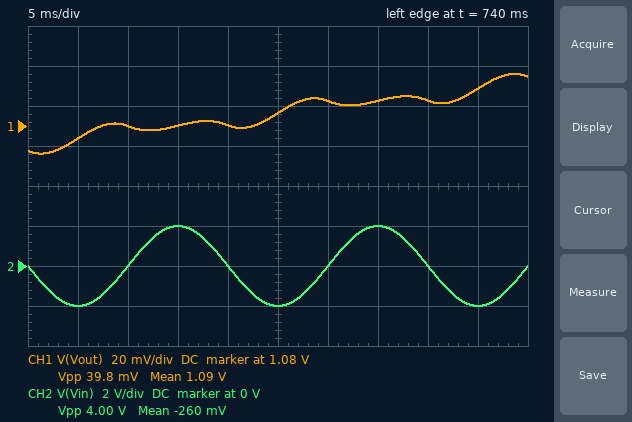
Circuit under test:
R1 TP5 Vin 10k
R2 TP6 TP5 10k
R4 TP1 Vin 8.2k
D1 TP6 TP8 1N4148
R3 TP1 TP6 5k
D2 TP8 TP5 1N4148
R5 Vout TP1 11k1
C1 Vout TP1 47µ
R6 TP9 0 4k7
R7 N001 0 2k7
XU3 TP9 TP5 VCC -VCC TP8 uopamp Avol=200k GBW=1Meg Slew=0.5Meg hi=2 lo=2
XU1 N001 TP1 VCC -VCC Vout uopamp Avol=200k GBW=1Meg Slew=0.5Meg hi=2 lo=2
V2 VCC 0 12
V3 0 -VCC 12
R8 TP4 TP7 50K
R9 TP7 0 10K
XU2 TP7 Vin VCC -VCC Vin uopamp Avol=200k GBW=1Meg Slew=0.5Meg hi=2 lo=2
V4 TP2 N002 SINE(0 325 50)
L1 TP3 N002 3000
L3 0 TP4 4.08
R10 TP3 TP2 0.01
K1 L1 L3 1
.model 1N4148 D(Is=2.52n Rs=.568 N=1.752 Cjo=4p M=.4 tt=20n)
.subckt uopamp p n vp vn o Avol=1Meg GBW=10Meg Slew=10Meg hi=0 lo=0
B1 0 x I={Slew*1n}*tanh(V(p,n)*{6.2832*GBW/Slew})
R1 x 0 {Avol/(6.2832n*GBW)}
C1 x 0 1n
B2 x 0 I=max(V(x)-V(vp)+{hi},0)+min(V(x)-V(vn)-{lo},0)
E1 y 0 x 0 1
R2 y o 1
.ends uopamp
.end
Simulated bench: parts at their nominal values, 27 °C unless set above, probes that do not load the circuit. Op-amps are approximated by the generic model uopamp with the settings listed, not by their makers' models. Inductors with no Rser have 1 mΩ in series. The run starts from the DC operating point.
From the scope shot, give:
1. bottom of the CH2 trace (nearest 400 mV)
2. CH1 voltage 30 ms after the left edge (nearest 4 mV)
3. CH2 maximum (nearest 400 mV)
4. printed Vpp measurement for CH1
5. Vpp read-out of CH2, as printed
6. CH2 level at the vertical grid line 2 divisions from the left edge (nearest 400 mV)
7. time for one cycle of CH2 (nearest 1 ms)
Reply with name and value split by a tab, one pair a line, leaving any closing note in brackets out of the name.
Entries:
bottom of the CH2 trace	-2.0 V
CH1 voltage 30 ms after the left edge	1.092 V
CH2 maximum	2.0 V
printed Vpp measurement for CH1	39.8 mV
Vpp read-out of CH2, as printed	4.00 V
CH2 level at the vertical grid line 2 divisions from the left edge	0 V
time for one cycle of CH2	20 ms
